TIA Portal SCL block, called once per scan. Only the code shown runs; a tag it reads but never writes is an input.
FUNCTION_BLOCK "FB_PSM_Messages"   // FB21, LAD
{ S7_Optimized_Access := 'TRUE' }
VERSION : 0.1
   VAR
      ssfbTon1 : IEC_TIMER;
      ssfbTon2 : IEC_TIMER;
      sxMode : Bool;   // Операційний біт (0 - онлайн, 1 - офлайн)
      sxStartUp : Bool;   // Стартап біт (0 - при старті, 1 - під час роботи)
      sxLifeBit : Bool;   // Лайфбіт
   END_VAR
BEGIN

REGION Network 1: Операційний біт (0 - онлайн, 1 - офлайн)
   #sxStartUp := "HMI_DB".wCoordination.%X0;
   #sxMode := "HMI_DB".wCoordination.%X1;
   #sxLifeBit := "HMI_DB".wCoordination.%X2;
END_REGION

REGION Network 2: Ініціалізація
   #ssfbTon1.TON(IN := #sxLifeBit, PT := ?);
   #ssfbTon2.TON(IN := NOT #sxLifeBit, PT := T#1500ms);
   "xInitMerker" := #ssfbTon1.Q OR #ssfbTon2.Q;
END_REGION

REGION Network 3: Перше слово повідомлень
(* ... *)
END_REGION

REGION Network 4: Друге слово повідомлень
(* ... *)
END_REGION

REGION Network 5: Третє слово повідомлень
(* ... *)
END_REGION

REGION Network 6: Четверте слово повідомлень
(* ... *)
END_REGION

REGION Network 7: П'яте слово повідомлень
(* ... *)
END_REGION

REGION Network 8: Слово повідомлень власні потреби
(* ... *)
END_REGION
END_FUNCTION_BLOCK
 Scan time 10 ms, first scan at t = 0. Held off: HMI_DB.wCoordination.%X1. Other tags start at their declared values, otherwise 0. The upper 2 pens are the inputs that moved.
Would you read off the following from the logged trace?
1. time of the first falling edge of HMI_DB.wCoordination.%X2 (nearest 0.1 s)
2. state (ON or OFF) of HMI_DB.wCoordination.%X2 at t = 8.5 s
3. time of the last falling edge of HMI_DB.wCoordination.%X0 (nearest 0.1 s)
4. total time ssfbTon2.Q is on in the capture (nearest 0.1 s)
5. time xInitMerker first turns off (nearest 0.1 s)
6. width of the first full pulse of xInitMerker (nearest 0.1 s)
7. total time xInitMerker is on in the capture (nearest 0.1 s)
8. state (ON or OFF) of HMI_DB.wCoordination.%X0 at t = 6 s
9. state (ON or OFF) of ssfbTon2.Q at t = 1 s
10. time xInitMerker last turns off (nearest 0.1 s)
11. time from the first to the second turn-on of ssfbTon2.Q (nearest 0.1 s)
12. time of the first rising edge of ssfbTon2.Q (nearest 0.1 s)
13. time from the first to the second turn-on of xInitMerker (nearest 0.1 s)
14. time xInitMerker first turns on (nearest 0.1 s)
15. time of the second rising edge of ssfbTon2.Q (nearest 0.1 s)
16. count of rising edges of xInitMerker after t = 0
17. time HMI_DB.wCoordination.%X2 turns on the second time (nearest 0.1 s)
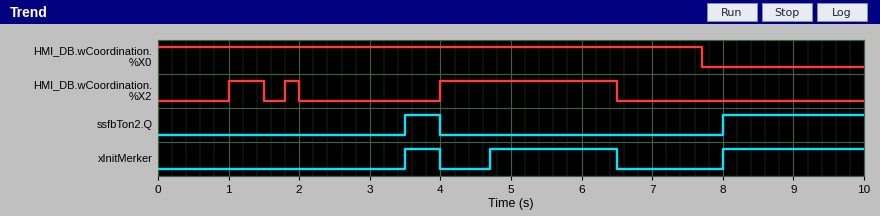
1.5 s
OFF
7.7 s
2.5 s
4.0 s
0.5 s
4.3 s
ON
OFF
6.5 s
4.5 s
3.5 s
1.2 s
3.5 s
8.0 s
3
1.8 s
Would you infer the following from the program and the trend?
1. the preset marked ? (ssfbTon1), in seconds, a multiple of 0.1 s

0.7 s
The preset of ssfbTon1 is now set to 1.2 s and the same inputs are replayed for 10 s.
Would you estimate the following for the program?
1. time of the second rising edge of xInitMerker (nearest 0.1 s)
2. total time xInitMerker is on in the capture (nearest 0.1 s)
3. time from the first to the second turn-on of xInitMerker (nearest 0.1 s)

5.2 s
3.8 s
1.7 s
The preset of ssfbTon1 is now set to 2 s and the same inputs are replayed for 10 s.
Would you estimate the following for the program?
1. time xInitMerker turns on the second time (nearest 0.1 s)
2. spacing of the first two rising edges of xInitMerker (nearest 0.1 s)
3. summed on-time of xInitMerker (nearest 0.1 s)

6.0 s
2.5 s
3.0 s
